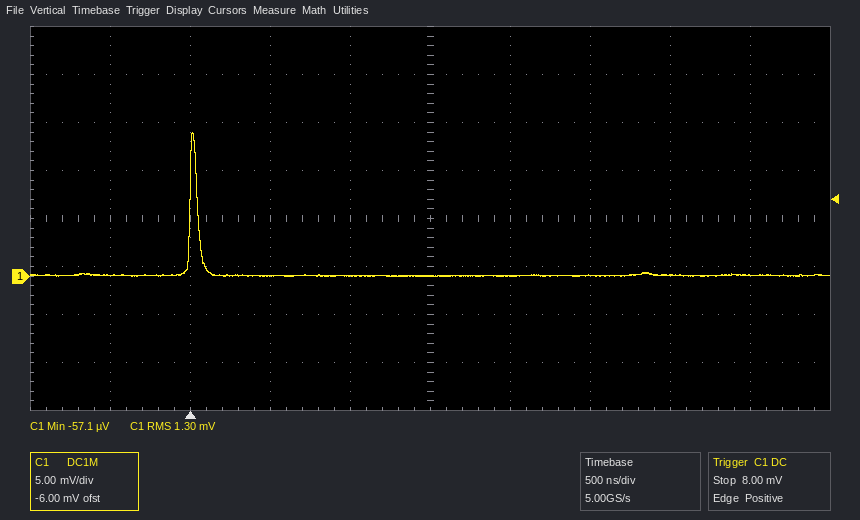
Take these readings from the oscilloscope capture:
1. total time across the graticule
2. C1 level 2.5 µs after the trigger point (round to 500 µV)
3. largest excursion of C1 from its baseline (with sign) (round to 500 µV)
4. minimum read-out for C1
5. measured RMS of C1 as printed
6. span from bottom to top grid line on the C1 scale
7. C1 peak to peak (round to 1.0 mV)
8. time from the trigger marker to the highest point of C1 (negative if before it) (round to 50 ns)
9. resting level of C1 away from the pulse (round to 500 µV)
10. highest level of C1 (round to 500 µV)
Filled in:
5 µs
0.0 mV
+15.0 mV
-57.1 µV
1.30 mV
40 mV
15.0 mV
0 ns
0.0 mV
15.0 mV
